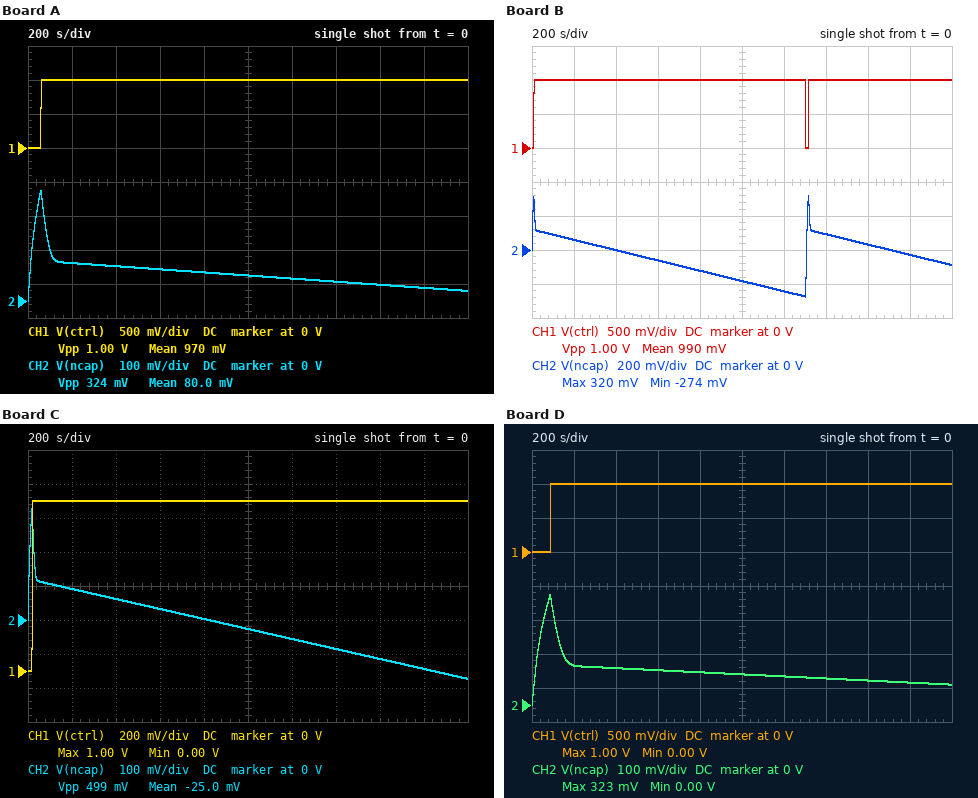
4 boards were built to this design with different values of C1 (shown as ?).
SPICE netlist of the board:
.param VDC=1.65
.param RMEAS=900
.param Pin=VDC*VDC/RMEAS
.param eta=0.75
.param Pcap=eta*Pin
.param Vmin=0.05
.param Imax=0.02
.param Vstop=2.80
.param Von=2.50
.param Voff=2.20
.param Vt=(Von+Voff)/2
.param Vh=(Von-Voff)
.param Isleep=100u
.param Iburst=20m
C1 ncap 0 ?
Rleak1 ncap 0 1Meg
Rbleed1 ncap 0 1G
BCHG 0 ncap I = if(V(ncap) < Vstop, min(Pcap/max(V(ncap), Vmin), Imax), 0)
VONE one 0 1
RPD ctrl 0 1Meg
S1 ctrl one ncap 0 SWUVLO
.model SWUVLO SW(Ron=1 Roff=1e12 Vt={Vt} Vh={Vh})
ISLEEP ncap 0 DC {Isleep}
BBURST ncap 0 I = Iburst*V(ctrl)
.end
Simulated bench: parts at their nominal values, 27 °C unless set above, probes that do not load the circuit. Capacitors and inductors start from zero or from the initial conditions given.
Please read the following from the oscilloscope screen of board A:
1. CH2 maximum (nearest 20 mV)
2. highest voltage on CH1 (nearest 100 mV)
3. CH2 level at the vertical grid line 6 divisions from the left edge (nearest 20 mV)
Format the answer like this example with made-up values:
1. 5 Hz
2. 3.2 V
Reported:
1. 320 mV
2. 1.0 V
3. 60 mV
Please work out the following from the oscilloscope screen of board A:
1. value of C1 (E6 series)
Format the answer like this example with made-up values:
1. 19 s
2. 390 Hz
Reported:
1. 2.2 F
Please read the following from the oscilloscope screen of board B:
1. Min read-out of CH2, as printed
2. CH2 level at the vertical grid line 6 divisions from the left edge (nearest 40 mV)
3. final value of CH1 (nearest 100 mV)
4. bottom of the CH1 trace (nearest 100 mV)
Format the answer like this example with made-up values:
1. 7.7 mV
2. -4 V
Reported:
1. -274 mV
2. -240 mV
3. 1.0 V
4. 0 V
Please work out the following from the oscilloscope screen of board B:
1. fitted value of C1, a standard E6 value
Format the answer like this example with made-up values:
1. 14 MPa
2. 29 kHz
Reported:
1. 330 mF
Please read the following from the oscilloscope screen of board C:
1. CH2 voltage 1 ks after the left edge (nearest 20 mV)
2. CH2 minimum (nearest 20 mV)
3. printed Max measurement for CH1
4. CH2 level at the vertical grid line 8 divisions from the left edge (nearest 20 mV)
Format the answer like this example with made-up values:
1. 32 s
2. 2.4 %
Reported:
1. -20 mV
2. -180 mV
3. 1.00 V
4. -120 mV
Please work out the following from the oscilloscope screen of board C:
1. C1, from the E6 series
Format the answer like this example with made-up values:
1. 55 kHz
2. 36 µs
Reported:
1. 680 mF
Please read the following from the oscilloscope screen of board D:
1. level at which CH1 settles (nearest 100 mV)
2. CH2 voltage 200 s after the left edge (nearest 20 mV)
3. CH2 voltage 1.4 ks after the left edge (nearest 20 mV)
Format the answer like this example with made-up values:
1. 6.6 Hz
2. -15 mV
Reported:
1. 1.0 V
2. 120 mV
3. 80 mV
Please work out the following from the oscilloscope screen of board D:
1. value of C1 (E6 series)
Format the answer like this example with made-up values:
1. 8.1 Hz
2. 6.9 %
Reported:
1. 3.3 F
